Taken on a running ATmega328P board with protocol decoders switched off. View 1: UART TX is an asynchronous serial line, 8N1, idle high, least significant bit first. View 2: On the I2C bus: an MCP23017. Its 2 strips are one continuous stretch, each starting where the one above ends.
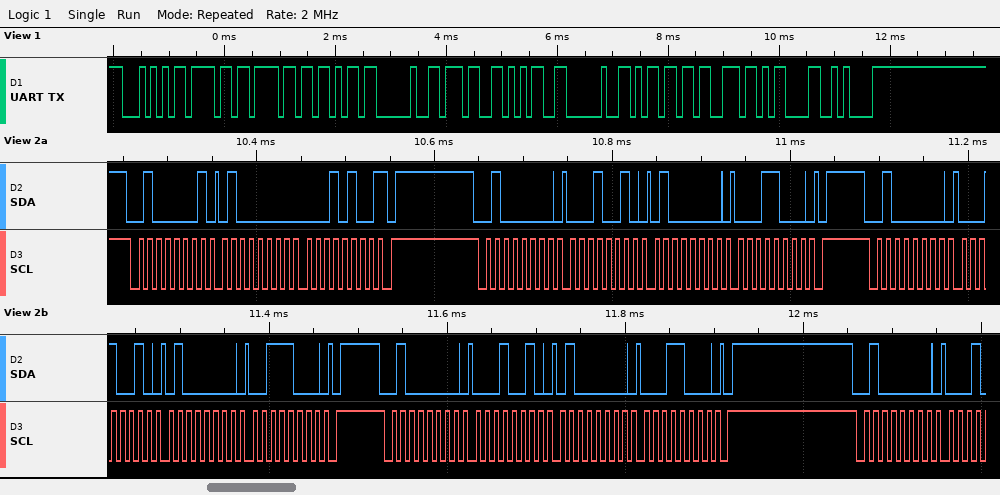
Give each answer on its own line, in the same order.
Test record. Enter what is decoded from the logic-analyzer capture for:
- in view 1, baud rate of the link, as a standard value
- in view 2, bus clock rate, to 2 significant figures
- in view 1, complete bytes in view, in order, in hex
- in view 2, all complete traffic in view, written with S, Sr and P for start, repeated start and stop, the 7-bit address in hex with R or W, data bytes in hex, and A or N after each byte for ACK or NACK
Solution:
9600 baud
100 kHz
54 6F 6F 6B 20 37 35 20 6D 73 0D 0A
S 20R A 40 A 14 N P S 20W A 12 A 40 A 18 A P S 20W A 12 A 40 A 38 A P S 20W A 12 A 40 A 18 A P S 20W A
